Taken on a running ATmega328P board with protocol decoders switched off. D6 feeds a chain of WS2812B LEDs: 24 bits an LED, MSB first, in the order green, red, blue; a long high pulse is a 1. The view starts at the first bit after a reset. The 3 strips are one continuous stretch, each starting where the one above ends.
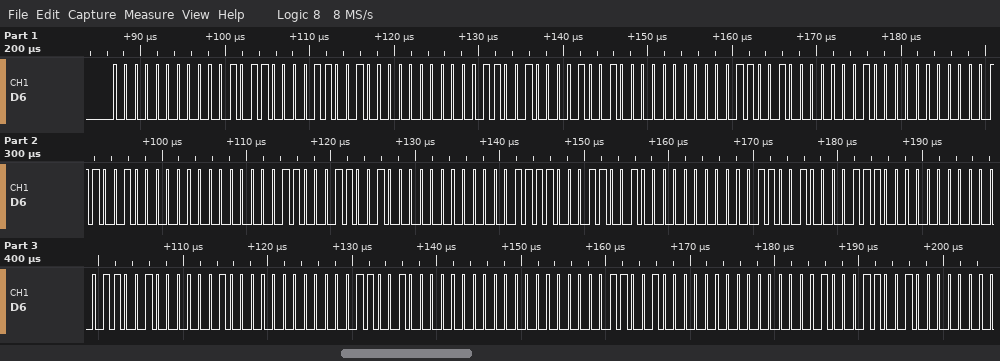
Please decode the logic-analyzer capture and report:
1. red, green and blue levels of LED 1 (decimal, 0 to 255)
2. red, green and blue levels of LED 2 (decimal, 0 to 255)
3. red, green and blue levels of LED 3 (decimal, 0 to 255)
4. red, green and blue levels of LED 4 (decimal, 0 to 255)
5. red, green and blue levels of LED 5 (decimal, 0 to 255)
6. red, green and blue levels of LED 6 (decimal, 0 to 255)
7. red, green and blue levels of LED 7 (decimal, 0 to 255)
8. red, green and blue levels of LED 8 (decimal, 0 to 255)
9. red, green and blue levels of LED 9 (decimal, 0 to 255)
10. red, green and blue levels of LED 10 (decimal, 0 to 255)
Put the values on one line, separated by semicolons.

22, 0, 25; 25, 0, 9; 25, 0, 1; 25, 0, 0; 25, 3, 0; 25, 15, 0; 14, 25, 0; 2, 25, 0; 0, 25, 0; 0, 25, 1
